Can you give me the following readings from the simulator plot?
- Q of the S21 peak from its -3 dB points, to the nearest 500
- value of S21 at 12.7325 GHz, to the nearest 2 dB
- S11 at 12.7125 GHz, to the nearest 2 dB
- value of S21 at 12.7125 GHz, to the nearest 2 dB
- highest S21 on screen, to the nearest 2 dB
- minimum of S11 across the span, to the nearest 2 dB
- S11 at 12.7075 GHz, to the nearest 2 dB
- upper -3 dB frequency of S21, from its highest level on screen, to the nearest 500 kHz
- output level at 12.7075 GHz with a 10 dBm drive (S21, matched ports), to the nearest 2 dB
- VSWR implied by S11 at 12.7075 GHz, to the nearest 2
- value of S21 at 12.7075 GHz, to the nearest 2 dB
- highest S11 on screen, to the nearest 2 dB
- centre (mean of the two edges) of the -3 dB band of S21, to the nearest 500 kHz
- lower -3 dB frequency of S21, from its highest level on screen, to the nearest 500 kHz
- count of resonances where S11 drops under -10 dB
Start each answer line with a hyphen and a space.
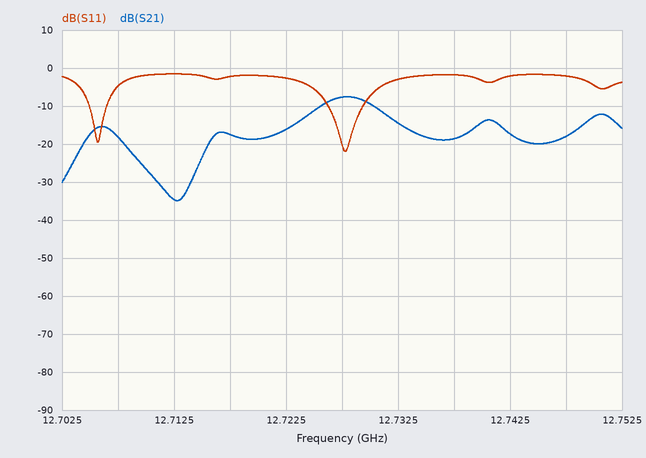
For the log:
- 2500
- -14 dB
- -2 dB
- -34 dB
- -8 dB
- -22 dB
- -4 dB
- 12.7305 GHz
- -8 dBm
- 4
- -18 dB
- -2 dB
- 12.7280 GHz
- 12.7255 GHz
- 2
